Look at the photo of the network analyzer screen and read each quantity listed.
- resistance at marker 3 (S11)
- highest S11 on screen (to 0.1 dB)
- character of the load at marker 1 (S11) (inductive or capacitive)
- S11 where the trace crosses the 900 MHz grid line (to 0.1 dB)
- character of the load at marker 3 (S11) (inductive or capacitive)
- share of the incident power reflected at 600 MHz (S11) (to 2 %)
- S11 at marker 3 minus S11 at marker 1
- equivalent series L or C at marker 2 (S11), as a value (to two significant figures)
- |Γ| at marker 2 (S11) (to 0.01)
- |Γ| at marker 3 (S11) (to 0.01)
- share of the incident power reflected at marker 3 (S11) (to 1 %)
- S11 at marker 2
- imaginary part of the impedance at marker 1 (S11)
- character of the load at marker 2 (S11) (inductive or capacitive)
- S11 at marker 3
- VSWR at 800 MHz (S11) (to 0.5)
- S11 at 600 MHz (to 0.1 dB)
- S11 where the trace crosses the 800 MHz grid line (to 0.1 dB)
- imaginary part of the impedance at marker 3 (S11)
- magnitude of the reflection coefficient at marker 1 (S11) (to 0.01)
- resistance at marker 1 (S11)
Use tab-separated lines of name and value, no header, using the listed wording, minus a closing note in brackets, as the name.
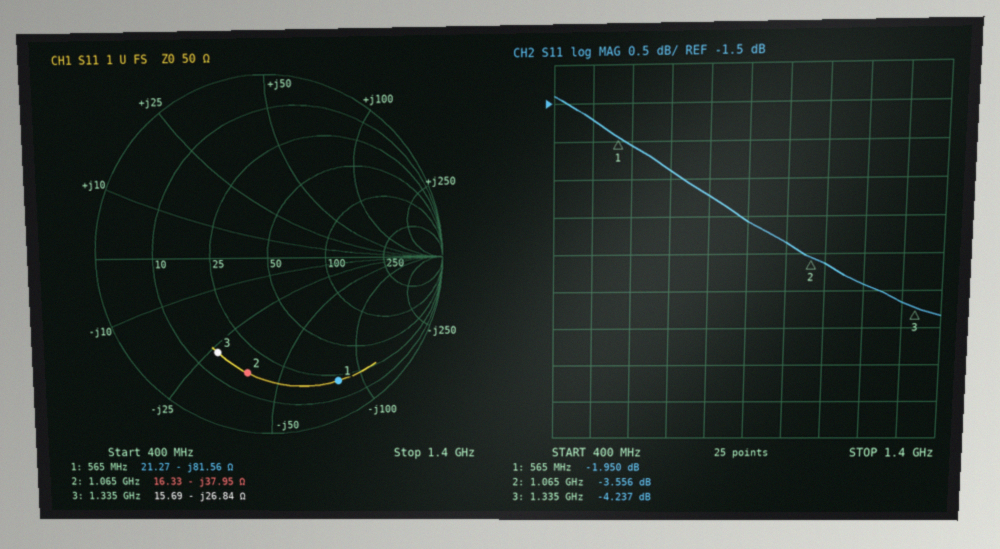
resistance at marker 3	15.69 Ω
highest S11 on screen	-1.4 dB
character of the load at marker 1 (S11)	capacitive
S11 where the trace crosses the 900 MHz grid line	-3.1 dB
character of the load at marker 3 (S11)	capacitive
share of the incident power reflected at 600 MHz (S11)	62 %
S11 at marker 3 minus S11 at marker 1	-2.287 dB
equivalent series L or C at marker 2 (S11), as a value	3.9 pF
|Γ| at marker 2 (S11)	0.66
|Γ| at marker 3 (S11)	0.61
share of the incident power reflected at marker 3 (S11)	38 %
S11 at marker 2	-3.556 dB
imaginary part of the impedance at marker 1	-81.56 Ω
character of the load at marker 2 (S11)	capacitive
S11 at marker 3	-4.237 dB
VSWR at 800 MHz (S11)	6.5
S11 at 600 MHz	-2.1 dB
S11 where the trace crosses the 800 MHz grid line	-2.7 dB
imaginary part of the impedance at marker 3	-26.84 Ω
magnitude of the reflection coefficient at marker 1 (S11)	0.80
resistance at marker 1	21.27 Ω
